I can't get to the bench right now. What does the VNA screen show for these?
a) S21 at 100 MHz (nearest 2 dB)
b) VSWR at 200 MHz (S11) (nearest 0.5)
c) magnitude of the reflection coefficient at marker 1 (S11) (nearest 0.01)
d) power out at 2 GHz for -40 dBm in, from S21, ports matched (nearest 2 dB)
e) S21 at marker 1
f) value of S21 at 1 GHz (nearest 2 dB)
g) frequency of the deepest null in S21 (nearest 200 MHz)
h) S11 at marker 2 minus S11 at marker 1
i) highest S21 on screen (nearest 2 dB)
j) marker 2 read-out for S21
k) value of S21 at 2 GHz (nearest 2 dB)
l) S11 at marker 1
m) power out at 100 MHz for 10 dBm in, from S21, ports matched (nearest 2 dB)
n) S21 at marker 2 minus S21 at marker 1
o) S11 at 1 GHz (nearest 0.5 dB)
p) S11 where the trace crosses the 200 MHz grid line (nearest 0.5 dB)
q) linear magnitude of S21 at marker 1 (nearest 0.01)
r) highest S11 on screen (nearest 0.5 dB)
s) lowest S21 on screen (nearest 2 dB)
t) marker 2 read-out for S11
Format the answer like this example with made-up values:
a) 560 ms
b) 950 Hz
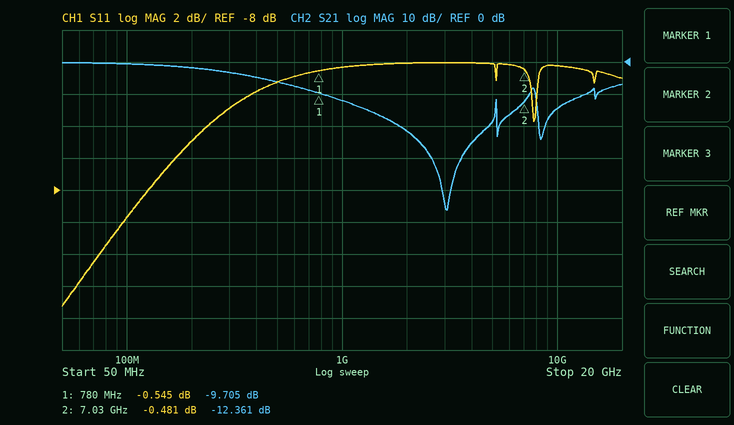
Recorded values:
a) 0 dB
b) 3.5
c) 0.94
d) -62 dBm
e) -9.705 dB
f) -12 dB
g) 3.0 GHz
h) 0.064 dB
i) 0 dB
j) -12.361 dB
k) -22 dB
l) -0.545 dB
m) 10 dBm
n) -2.656 dB
o) -0.5 dB
p) -5.0 dB
q) 0.33
r) 0.0 dB
s) -46 dB
t) -0.481 dB
